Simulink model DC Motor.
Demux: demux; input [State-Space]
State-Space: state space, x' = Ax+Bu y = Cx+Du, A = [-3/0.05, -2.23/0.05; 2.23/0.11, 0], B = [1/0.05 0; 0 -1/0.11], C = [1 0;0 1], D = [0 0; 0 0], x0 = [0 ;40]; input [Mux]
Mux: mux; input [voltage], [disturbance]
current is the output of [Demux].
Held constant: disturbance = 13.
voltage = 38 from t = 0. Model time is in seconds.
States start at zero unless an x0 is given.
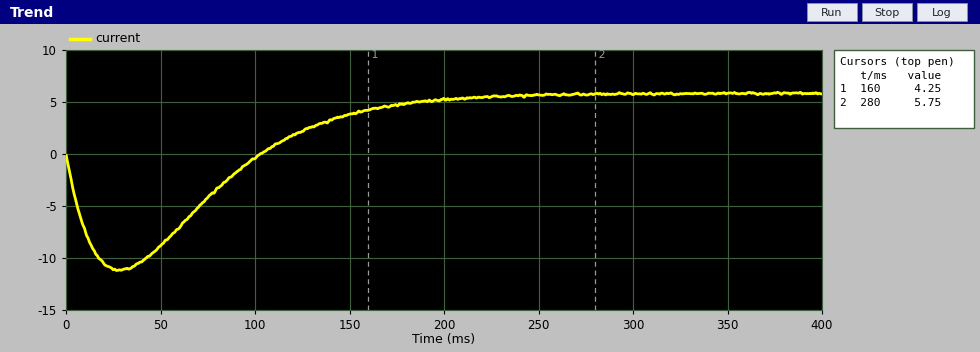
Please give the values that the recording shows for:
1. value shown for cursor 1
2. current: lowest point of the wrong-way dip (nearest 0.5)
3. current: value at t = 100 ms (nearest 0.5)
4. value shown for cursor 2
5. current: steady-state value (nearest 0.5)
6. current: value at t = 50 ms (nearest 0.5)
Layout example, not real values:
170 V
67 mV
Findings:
4.25
-11.0
-0.5
5.75
6.0
-9.0
